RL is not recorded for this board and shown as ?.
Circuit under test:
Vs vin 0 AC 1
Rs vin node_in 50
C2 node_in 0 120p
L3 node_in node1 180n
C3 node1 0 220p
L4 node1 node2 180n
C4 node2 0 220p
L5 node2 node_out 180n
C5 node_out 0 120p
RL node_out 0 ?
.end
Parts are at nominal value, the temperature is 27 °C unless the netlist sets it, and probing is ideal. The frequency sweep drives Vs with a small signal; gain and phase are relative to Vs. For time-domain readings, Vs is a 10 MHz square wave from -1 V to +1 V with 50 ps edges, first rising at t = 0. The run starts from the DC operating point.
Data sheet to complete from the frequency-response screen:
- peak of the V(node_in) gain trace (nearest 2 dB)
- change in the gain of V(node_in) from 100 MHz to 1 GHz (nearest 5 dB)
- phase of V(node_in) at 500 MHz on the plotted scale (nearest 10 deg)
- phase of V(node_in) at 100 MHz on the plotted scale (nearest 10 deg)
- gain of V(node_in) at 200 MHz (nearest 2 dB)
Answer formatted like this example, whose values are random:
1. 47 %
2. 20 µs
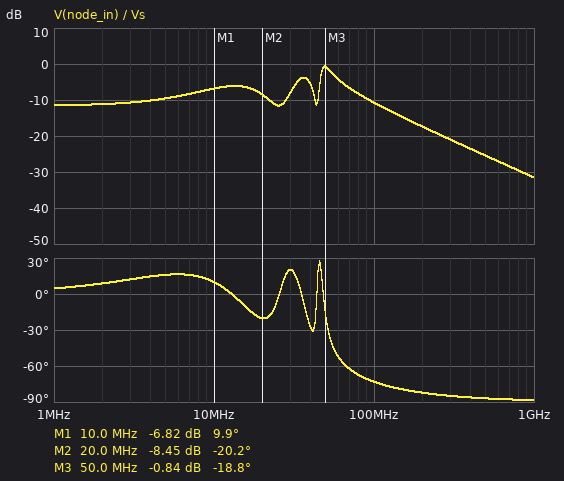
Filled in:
1. 0 dB
2. -20 dB
3. -90 deg
4. -70 deg
5. -18 dB
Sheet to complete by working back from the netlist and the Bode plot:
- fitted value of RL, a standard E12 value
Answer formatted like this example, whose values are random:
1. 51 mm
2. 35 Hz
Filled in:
1. 18 Ω
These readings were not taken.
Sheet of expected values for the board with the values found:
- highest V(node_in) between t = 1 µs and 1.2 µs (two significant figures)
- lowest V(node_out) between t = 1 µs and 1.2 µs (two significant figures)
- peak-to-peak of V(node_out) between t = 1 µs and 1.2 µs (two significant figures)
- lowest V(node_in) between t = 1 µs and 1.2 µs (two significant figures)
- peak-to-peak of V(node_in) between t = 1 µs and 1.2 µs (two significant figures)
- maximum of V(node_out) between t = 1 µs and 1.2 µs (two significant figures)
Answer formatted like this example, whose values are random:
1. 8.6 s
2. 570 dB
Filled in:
1. 810 mV
2. -400 mV
3. 800 mV
4. -810 mV
5. 1.6 V
6. 400 mV
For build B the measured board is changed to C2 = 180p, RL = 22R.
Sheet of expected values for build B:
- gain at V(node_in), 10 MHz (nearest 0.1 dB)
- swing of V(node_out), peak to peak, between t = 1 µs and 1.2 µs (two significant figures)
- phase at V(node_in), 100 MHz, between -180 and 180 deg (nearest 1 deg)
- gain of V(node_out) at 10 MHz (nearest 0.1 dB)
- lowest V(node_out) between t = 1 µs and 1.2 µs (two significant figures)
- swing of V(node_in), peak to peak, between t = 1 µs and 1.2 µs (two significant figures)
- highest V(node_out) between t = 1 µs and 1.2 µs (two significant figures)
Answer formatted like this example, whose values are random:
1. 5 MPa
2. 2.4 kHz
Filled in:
1. -7.5 dB
2. 880 mV
3. -79 deg
4. -9.7 dB
5. -440 mV
6. 1.2 V
7. 440 mV
